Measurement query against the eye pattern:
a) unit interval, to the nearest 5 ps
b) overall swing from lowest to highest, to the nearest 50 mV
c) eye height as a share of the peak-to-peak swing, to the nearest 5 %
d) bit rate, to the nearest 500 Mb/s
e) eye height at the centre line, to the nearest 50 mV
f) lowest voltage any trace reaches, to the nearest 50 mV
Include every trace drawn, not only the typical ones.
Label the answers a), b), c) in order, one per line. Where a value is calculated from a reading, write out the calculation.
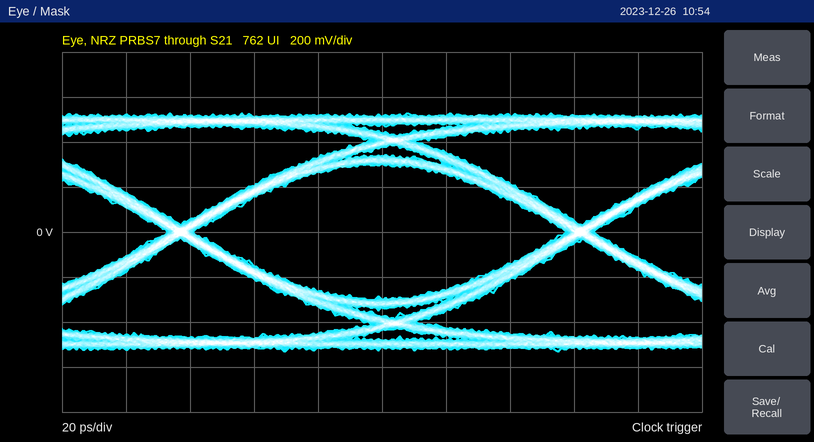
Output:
a) 125 ps
b) 1.05 V
c) 600 mV / 1.05 V ≈ 57.1 %, so 55 % to the nearest 5 %
d) 8.0 Gb/s
e) 600 mV
f) -550 mV
